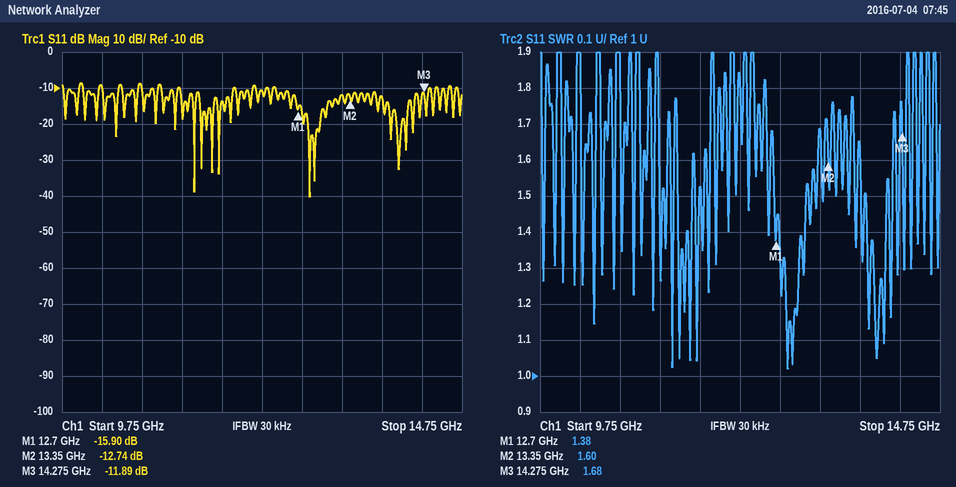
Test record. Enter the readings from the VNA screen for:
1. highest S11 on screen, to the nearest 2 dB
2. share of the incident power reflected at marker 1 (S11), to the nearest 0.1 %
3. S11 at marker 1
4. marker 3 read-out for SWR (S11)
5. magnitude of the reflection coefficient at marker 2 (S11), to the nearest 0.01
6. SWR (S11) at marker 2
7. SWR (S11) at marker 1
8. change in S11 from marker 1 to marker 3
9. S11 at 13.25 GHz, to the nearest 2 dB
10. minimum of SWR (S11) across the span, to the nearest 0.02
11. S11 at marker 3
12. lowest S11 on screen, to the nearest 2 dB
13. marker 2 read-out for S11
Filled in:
-8 dB
2.6 %
-15.90 dB
1.68
0.23
1.60
1.38
4.01 dB
-12 dB
1.02
-11.89 dB
-40 dB
-12.74 dB
